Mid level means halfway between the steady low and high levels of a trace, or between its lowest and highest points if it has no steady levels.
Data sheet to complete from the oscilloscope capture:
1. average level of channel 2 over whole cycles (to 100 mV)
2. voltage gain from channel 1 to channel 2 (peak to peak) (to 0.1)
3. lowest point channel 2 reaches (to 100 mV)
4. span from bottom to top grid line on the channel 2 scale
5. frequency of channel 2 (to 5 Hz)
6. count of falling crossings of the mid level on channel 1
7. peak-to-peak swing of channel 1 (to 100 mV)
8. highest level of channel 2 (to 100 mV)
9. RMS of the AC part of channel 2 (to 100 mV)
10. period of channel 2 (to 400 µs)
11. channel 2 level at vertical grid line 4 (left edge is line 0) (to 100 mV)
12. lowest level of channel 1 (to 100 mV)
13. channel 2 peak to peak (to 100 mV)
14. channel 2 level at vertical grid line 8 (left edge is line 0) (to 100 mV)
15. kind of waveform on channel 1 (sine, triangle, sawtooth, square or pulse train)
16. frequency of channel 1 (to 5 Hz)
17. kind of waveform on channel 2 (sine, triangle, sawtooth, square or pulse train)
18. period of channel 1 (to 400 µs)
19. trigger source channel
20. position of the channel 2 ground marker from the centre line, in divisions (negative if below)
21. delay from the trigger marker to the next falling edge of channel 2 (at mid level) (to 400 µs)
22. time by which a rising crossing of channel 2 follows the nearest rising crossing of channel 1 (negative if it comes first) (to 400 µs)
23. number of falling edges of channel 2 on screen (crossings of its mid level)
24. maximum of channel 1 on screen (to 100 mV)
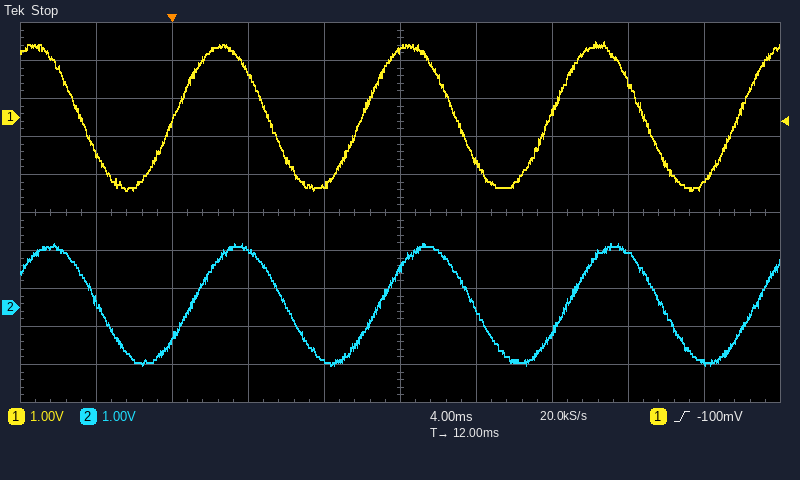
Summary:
100 mV
0.8
-1.5 V
10 V
100 Hz
4
3.9 V
1.7 V
1.1 V
10.0 ms
-1.4 V
-1.9 V
3.2 V
1.4 V
sine
100 Hz
sine
10.0 ms
channel 1
-2.5 div
6.0 ms
+800 µs
4
2.0 V
